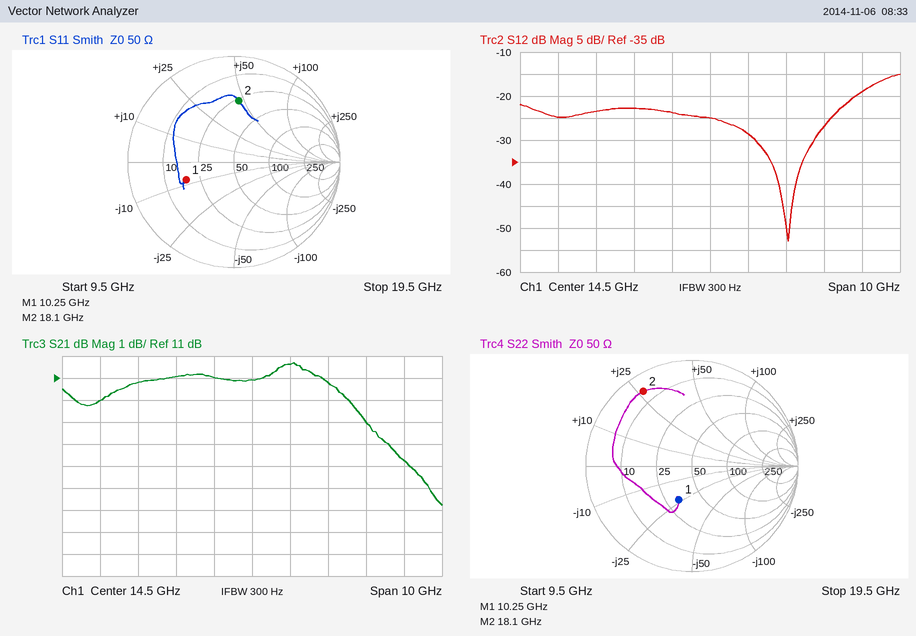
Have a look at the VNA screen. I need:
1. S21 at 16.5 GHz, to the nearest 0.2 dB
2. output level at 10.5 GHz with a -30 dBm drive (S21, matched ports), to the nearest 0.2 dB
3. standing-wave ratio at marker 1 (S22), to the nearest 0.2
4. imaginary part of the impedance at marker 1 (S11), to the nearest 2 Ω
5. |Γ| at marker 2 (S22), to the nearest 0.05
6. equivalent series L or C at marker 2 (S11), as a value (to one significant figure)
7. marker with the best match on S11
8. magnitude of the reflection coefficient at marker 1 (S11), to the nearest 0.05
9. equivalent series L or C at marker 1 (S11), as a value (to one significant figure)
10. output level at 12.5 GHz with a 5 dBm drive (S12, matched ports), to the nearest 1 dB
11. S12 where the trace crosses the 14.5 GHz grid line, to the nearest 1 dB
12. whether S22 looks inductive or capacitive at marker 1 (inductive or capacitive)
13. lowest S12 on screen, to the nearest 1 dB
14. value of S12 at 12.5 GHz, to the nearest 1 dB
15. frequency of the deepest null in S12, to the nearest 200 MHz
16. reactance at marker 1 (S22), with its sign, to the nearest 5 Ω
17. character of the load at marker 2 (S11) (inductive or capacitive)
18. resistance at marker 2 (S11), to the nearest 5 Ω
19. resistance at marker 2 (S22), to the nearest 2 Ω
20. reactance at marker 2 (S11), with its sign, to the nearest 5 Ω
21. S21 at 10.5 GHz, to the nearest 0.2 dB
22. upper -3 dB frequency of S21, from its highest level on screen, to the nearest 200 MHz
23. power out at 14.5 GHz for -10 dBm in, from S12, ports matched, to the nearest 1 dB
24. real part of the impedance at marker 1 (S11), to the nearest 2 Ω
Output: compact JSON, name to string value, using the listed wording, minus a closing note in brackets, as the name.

{"S21 at 16.5 GHz, to the nearest 0.2 dB": "10.8 dB", "output level at 10.5 GHz with a -30 dBm drive (S21, matched ports), to the nearest 0.2 dB": "-20.0 dBm", "standing-wave ratio at marker 1 (S22), to the nearest 0.2": "2.0", "imaginary part of the impedance at marker 1 (S11), to the nearest 2 Ω": "-8 Ω", "|Γ| at marker 2 (S22), to the nearest 0.05": "0.85", "equivalent series L or C at marker 2 (S11), as a value": "400 pH", "marker with the best match on S11": "marker 1", "magnitude of the reflection coefficient at marker 1 (S11), to the nearest 0.05": "0.50", "equivalent series L or C at marker 1 (S11), as a value": "2 pF", "output level at 12.5 GHz with a 5 dBm drive (S12, matched ports), to the nearest 1 dB": "-18 dBm", "S12 where the trace crosses the 14.5 GHz grid line, to the nearest 1 dB": "-25 dB", "whether S22 looks inductive or capacitive at marker 1": "capacitive", "lowest S12 on screen, to the nearest 1 dB": "-53 dB", "value of S12 at 12.5 GHz, to the nearest 1 dB": "-23 dB", "frequency of the deepest null in S12, to the nearest 200 MHz": "16.6 GHz", "reactance at marker 1 (S22), with its sign, to the nearest 5 Ω": "-25 Ω", "character of the load at marker 2 (S11)": "inductive", "resistance at marker 2 (S11), to the nearest 5 Ω": "25 Ω", "resistance at marker 2 (S22), to the nearest 2 Ω": "6 Ω", "reactance at marker 2 (S11), with its sign, to the nearest 5 Ω": "+45 Ω", "S21 at 10.5 GHz, to the nearest 0.2 dB": "10.0 dB", "upper -3 dB frequency of S21, from its highest level on screen, to the nearest 200 MHz": "17.6 GHz", "power out at 14.5 GHz for -10 dBm in, from S12, ports matched, to the nearest 1 dB": "-35 dBm", "real part of the impedance at marker 1 (S11), to the nearest 2 Ω": "18 Ω"}
